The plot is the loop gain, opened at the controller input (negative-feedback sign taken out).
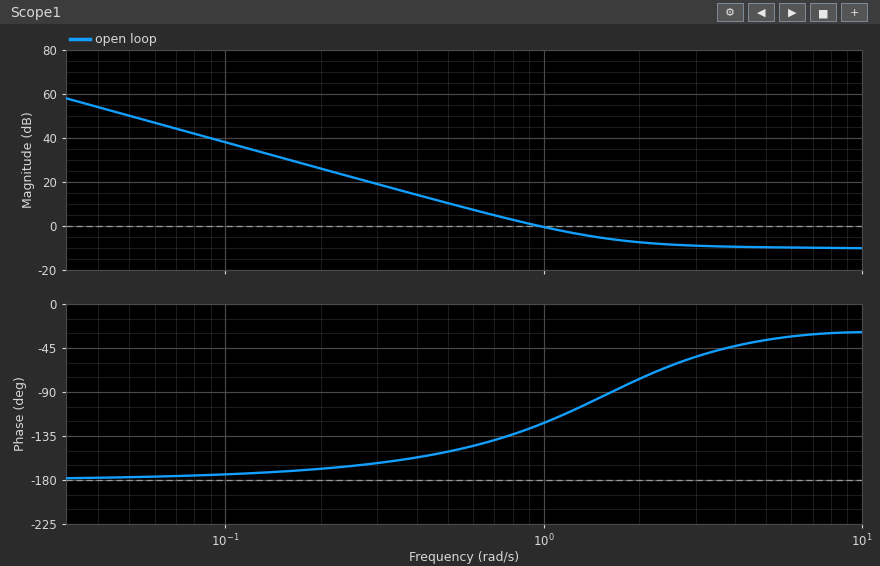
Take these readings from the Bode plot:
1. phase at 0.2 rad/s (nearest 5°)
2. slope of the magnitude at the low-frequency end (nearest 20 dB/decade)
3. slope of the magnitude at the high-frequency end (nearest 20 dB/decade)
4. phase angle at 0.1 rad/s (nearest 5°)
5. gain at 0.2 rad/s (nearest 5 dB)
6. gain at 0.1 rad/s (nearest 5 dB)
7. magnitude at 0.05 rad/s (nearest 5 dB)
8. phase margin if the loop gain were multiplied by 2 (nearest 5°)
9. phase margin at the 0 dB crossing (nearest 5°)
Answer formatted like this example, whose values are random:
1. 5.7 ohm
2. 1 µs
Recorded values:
1. -170°
2. -40 dB/decade
3. 0 dB/decade
4. -175°
5. 25 dB
6. 40 dB
7. 50 dB
8. 90°
9. 55°
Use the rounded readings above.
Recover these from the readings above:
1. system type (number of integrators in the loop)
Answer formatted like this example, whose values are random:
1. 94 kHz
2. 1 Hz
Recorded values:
1. 2
